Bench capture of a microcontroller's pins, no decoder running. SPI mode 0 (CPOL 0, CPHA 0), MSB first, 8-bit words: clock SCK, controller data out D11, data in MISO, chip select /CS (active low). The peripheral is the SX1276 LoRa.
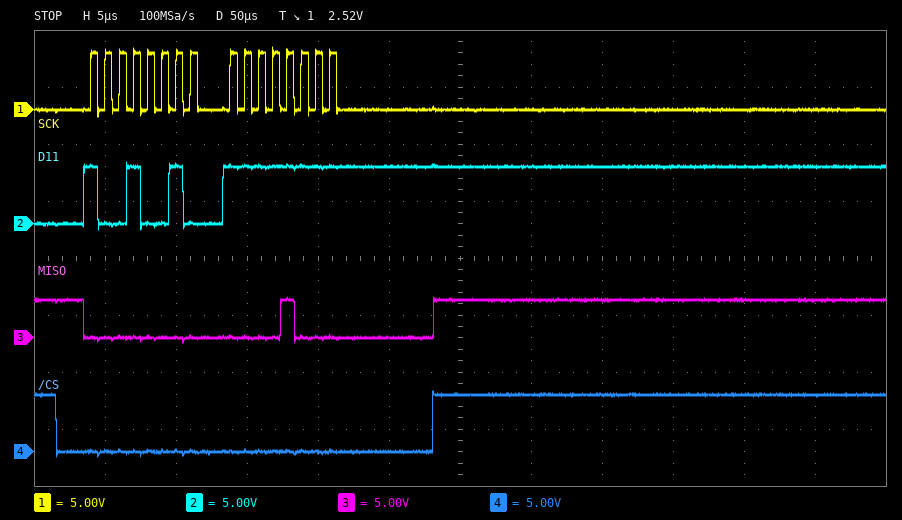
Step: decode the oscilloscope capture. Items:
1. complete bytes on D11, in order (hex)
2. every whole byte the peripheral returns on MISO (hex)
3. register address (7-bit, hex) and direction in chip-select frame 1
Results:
0x92 0xFF
0x00 0x08
0x12 write
